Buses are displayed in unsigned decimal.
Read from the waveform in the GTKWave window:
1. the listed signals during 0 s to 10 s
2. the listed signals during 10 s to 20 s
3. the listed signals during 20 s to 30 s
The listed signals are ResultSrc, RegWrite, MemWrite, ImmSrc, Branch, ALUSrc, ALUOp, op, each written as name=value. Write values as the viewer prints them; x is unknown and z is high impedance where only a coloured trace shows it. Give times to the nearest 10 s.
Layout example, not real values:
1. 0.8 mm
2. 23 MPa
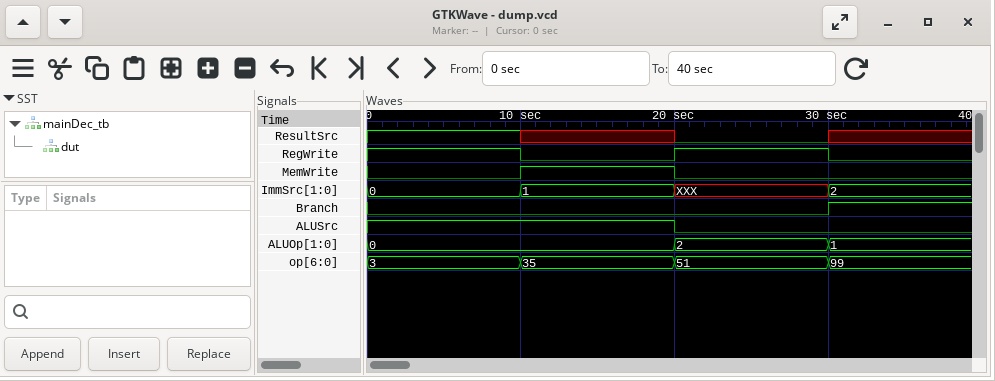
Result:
1. ResultSrc=1, RegWrite=1, MemWrite=0, ImmSrc=0, Branch=0, ALUSrc=1, ALUOp=0, op=3
2. ResultSrc=x, RegWrite=0, MemWrite=1, ImmSrc=1, Branch=0, ALUSrc=1, ALUOp=0, op=35
3. ResultSrc=0, RegWrite=1, MemWrite=0, ImmSrc=XXX, Branch=0, ALUSrc=0, ALUOp=2, op=51
